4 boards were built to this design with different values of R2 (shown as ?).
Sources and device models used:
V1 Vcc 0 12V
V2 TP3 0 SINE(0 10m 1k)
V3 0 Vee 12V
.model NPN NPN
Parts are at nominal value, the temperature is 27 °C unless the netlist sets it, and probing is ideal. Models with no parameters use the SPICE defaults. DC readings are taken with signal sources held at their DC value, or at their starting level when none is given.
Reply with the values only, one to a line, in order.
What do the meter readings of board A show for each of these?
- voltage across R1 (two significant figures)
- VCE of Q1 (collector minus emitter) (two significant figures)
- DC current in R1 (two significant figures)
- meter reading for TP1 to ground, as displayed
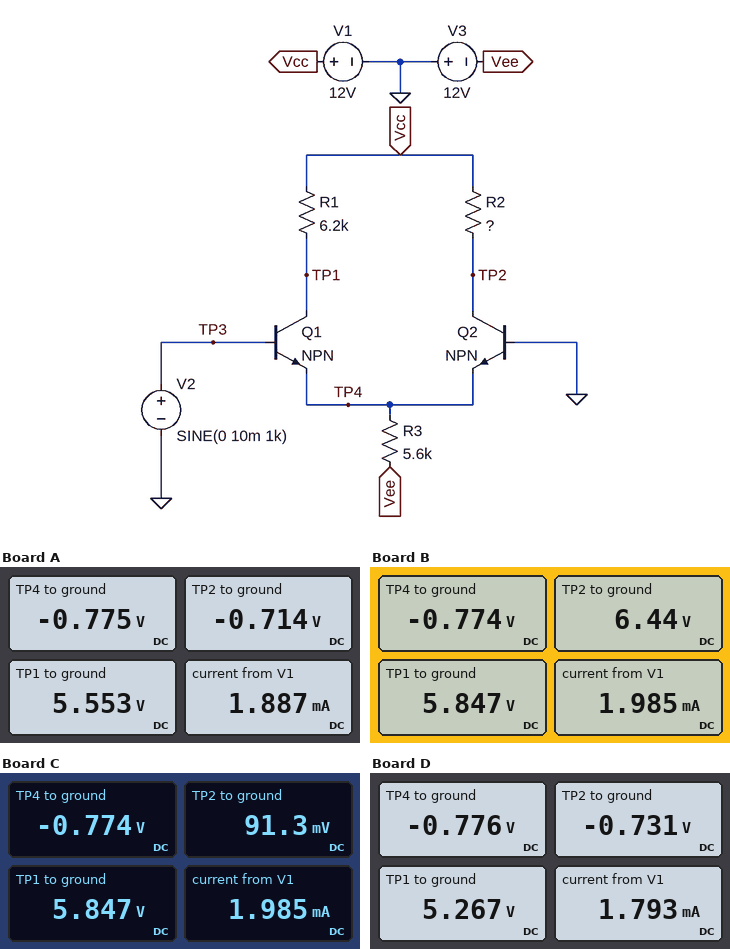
6.4 V
6.3 V
1.0 mA
5.553 V
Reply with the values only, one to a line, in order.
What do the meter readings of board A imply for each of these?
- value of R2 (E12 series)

15 kΩ
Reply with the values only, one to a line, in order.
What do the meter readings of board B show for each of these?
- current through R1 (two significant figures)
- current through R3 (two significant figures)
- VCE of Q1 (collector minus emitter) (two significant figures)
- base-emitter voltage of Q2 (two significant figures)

990 µA
2.0 mA
6.6 V
770 mV
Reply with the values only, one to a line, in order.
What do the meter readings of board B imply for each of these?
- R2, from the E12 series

5.6 kΩ
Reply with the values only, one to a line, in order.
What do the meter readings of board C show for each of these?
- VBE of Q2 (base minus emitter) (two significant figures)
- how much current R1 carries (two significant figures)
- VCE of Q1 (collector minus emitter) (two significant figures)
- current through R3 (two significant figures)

770 mV
990 µA
6.6 V
2.0 mA
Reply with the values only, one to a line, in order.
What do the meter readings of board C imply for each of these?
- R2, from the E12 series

12 kΩ
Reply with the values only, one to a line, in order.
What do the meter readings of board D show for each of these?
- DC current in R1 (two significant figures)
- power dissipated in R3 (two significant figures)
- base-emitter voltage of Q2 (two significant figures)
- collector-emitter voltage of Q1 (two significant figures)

1.1 mA
22 mW
780 mV
6.0 V
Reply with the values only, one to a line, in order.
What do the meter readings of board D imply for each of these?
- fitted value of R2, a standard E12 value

18 kΩ
